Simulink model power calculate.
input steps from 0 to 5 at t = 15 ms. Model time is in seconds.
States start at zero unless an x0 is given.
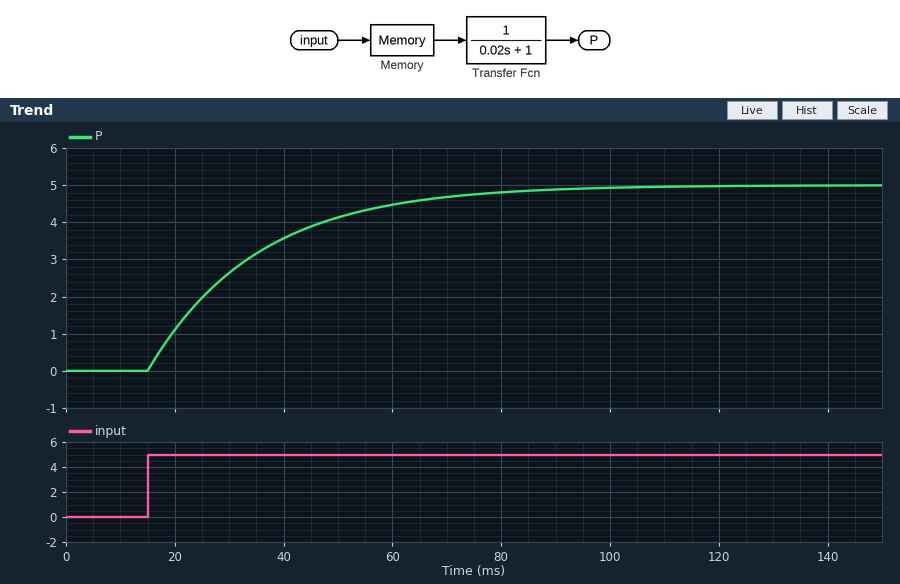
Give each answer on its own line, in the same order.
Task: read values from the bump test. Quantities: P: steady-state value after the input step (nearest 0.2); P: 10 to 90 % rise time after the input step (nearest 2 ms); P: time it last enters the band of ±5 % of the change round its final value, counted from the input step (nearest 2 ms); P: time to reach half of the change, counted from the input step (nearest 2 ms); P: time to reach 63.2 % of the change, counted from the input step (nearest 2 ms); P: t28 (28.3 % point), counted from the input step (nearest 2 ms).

5.0
44 ms
60 ms
14 ms
20 ms
6 ms
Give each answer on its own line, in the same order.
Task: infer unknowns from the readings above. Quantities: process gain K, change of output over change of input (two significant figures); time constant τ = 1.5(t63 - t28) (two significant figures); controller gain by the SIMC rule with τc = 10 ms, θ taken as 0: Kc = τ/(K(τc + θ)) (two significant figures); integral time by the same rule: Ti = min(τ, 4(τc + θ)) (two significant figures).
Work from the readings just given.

1.0
21 ms
2.1
21 ms
